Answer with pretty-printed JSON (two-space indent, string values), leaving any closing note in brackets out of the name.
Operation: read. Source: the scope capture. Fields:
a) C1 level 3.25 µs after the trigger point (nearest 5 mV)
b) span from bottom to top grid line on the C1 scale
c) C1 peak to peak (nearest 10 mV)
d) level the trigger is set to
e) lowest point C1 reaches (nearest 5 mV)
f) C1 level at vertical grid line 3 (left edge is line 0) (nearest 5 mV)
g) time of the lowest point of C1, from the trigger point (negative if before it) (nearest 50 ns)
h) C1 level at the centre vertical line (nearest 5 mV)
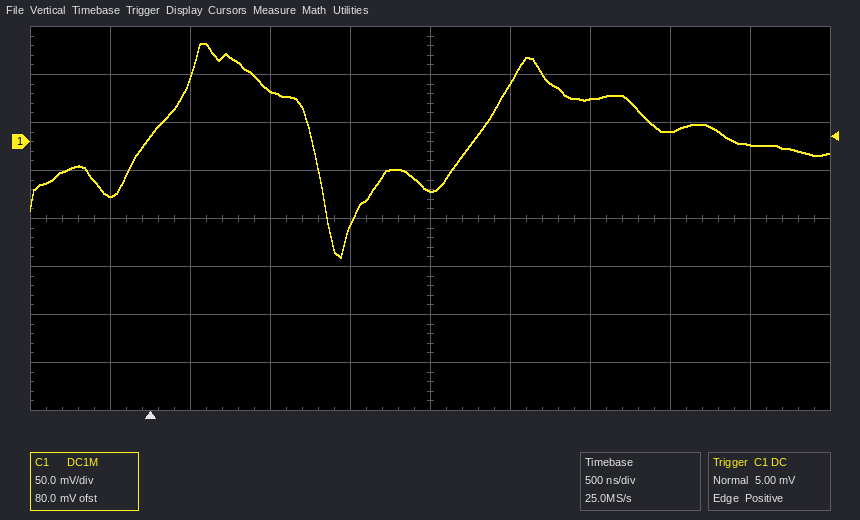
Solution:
{
  "C1 level 3.25 µs after the trigger point": "10 mV",
  "span from bottom to top grid line on the C1 scale": "400 mV",
  "C1 peak to peak": "220 mV",
  "level the trigger is set to": "5.00 mV",
  "lowest point C1 reaches": "-120 mV",
  "C1 level at vertical grid line 3 (left edge is line 0)": "55 mV",
  "time of the lowest point of C1, from the trigger point (negative if before it)": "+1.20 µs",
  "C1 level at the centre vertical line": "-50 mV"
}
